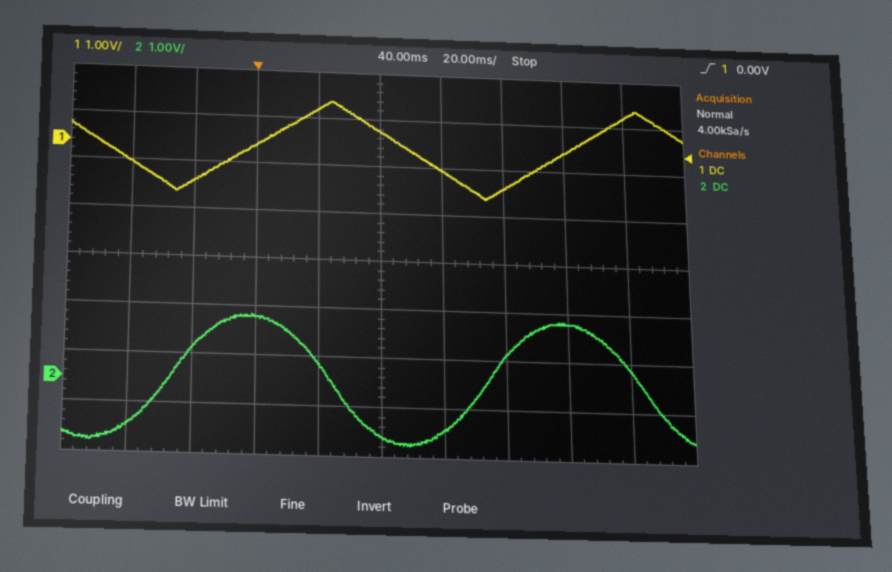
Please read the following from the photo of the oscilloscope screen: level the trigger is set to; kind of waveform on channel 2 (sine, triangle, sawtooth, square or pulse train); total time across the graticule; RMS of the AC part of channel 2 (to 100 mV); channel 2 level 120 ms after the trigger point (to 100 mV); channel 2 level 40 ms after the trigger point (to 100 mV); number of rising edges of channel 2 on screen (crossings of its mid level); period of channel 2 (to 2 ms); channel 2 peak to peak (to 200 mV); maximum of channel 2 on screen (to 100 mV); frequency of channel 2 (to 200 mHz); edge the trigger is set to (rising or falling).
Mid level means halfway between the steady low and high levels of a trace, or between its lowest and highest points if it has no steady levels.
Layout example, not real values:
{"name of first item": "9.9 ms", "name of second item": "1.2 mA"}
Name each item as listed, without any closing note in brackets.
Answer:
{"level the trigger is set to": "0.00 V", "kind of waveform on channel 2": "sine", "total time across the graticule": "200 ms", "RMS of the AC part of channel 2": "900 mV", "channel 2 level 120 ms after the trigger point": "400 mV", "channel 2 level 40 ms after the trigger point": "-1.1 V", "number of rising edges of channel 2 on screen": "2", "period of channel 2": "100 ms", "channel 2 peak to peak": "2.6 V", "maximum of channel 2 on screen": "1.3 V", "frequency of channel 2": "10.0 Hz", "edge the trigger is set to": "rising"}
